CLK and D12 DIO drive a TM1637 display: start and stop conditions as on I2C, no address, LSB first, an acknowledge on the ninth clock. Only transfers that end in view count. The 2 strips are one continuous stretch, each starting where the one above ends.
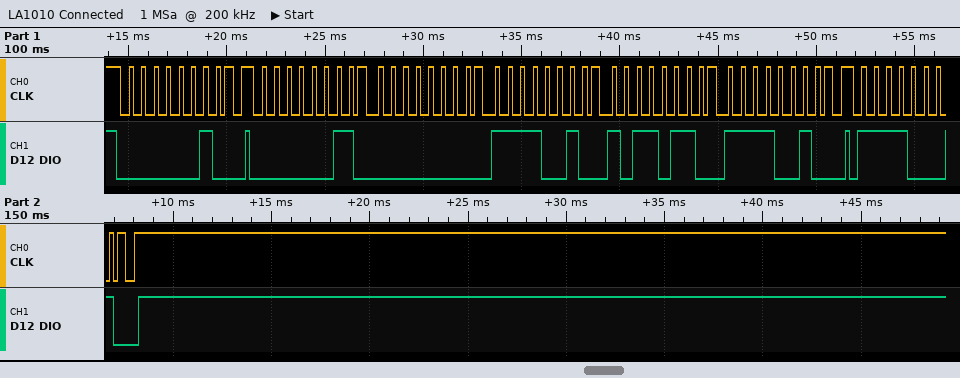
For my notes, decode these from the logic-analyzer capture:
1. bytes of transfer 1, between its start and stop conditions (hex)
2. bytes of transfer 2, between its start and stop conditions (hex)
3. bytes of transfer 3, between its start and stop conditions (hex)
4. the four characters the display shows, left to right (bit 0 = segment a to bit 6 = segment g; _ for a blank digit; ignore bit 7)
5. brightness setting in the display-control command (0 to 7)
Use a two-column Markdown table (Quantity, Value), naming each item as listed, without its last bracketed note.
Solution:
| Quantity | Value |
|---|---|
| bytes of transfer 1, between its start and stop conditions | 40 |
| bytes of transfer 2, between its start and stop conditions | C0 00 4F 6D 4F |
| bytes of transfer 3, between its start and stop conditions | 8F |
| the four characters the display shows, left to right | _353 |
| brightness setting in the display-control command | 7 |
